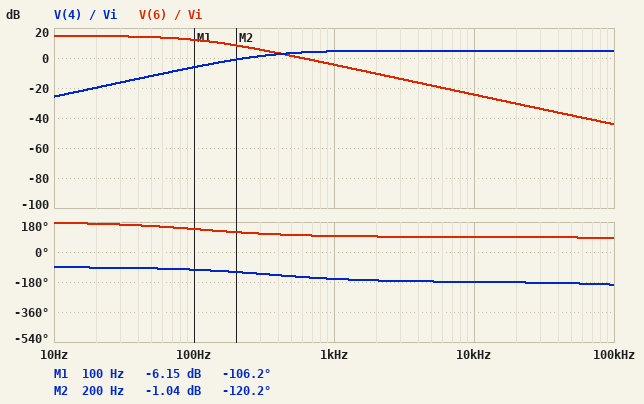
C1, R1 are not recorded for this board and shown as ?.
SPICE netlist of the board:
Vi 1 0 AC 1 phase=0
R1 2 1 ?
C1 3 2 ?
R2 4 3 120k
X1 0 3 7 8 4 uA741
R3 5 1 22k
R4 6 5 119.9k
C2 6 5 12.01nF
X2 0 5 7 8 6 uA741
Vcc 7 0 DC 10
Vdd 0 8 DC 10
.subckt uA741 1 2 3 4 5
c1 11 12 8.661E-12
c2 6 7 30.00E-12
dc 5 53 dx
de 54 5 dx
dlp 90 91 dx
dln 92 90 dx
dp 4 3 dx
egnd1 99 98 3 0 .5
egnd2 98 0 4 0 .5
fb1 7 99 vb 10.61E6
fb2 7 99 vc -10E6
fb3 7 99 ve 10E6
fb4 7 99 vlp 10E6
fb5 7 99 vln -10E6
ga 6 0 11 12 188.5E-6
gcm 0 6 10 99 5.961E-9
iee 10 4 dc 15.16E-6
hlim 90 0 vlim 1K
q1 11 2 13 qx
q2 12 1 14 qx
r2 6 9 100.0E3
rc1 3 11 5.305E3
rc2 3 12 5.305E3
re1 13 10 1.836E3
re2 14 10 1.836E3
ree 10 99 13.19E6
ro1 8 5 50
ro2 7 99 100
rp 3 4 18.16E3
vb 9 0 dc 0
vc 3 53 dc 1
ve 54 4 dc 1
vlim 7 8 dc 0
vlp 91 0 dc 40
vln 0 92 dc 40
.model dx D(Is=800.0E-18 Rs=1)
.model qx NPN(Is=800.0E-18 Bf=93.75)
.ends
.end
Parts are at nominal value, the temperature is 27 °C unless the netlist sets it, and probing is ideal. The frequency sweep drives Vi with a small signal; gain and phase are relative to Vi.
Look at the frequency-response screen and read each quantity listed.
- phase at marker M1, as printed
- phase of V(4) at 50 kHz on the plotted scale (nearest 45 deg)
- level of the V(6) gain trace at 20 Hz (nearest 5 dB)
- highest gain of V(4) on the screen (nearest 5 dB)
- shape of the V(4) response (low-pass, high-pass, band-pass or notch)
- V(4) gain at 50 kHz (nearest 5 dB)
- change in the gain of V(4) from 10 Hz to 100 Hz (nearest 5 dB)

-106.2 deg
-180 deg
15 dB
5 dB
high-pass
5 dB
20 dB
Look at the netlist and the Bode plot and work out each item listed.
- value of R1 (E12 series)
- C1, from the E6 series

68 kΩ
6.8 nF
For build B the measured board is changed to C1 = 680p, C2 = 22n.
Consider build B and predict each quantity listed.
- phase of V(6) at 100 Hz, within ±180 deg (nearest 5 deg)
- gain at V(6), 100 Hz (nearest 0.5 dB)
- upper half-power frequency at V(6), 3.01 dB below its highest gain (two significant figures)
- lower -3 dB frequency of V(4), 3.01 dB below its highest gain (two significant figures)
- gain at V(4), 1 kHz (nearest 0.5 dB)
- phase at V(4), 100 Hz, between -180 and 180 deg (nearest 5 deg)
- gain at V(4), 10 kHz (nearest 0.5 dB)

120 deg
9.0 dB
60 Hz
3.4 kHz
-6.0 dB
-90 deg
4.5 dB
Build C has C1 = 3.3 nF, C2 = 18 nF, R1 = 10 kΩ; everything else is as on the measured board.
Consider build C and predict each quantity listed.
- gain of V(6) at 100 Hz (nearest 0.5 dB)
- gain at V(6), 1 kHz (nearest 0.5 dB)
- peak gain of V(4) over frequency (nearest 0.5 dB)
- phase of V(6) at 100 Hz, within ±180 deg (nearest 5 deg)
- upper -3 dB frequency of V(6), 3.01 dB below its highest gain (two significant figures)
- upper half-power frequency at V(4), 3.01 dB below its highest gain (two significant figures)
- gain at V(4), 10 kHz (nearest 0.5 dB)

10.0 dB
-8.0 dB
21.5 dB
125 deg
74 Hz
84 kHz
21.0 dB
